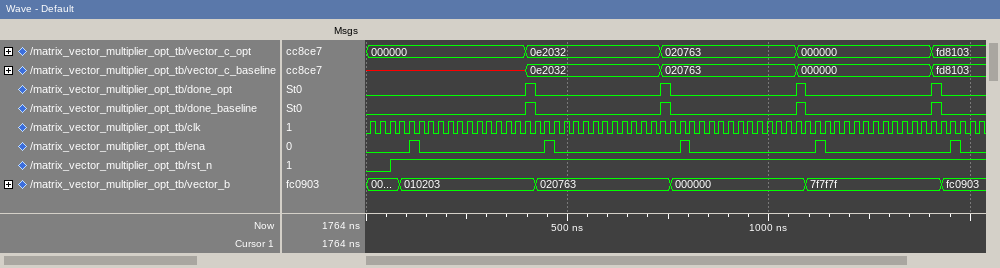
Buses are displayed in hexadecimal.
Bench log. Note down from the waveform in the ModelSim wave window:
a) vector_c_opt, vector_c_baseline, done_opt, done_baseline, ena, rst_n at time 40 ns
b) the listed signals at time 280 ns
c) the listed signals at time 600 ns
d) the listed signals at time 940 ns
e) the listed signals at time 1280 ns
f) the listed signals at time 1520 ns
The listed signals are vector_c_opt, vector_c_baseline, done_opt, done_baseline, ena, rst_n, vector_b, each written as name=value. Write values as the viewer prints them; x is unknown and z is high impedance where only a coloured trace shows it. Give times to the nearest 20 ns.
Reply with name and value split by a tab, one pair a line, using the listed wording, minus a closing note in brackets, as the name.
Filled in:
vector_c_opt, vector_c_baseline, done_opt, done_baseline, ena, rst_n at time 40 ns	vector_c_opt=000000, vector_c_baseline=x, done_opt=0, done_baseline=0, ena=0, rst_n=0
the listed signals at time 280 ns	vector_c_opt=000000, vector_c_baseline=x, done_opt=0, done_baseline=0, ena=0, rst_n=1, vector_b=010203
the listed signals at time 600 ns	vector_c_opt=0e2032, vector_c_baseline=0e2032, done_opt=0, done_baseline=0, ena=0, rst_n=1, vector_b=020763
the listed signals at time 940 ns	vector_c_opt=020763, vector_c_baseline=020763, done_opt=0, done_baseline=0, ena=0, rst_n=1, vector_b=000000
the listed signals at time 1280 ns	vector_c_opt=000000, vector_c_baseline=000000, done_opt=0, done_baseline=0, ena=0, rst_n=1, vector_b=7f7f7f
the listed signals at time 1520 ns	vector_c_opt=fd8103, vector_c_baseline=fd8103, done_opt=0, done_baseline=0, ena=0, rst_n=1, vector_b=fc0903
